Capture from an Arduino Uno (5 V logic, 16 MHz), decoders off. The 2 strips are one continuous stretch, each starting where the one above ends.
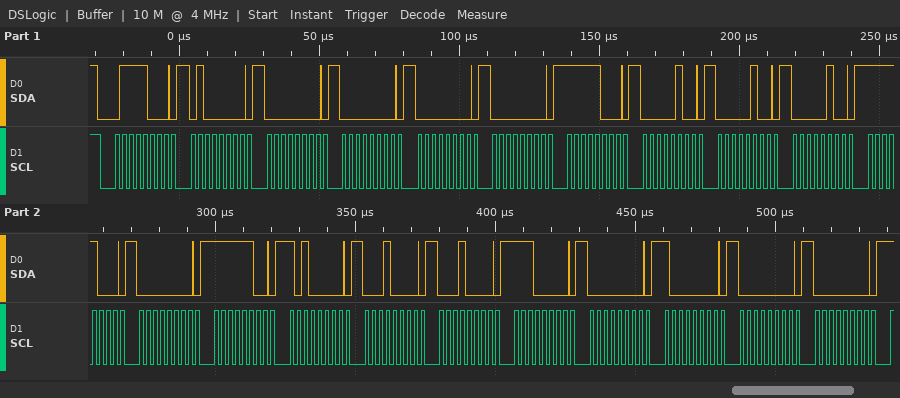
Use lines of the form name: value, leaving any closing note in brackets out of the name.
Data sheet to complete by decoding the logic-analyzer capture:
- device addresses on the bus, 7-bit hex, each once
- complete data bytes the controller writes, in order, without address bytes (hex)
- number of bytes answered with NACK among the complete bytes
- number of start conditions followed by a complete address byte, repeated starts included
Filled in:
device addresses on the bus, 7-bit hex, each once: 0x3C
complete data bytes the controller writes, in order, without address bytes: 40 00 00 00 00 F8 04 04 04 F8 00 FC A0 10 10 E0 00 80 00 00
number of bytes answered with NACK among the complete bytes: 0
number of start conditions followed by a complete address byte, repeated starts included: 1
